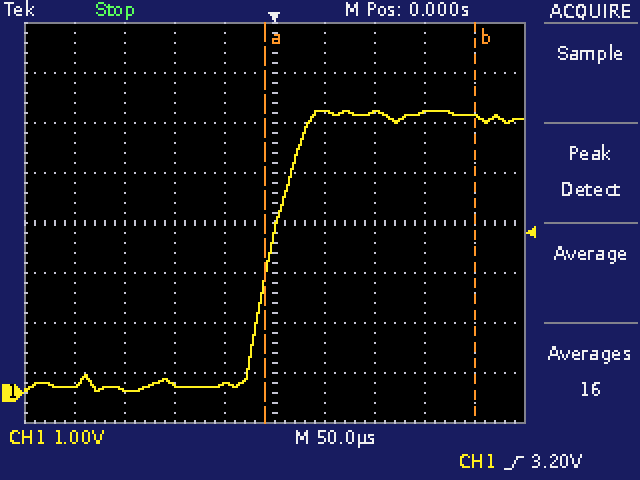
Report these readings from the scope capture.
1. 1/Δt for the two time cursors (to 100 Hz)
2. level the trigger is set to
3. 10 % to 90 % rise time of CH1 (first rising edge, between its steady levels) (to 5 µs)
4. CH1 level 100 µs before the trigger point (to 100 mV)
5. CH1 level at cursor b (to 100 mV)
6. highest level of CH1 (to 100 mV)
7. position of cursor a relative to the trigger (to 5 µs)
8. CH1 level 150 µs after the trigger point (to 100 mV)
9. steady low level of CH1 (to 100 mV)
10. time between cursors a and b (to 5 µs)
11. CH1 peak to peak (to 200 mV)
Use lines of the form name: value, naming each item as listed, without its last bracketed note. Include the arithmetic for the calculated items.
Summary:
1/Δt for the two time cursors: 1 / 210 µs ≈ 4.8 kHz
level the trigger is set to: 3.20 V
10 % to 90 % rise time of CH1 (first rising edge, between its steady levels): 50 µs
CH1 level 100 µs before the trigger point: 200 mV
CH1 level at cursor b: 5.5 V
highest level of CH1: 5.6 V
position of cursor a relative to the trigger: -10 µs
CH1 level 150 µs after the trigger point: 5.6 V
steady low level of CH1: 100 mV
time between cursors a and b: 210 µs
CH1 peak to peak: 5.6 V
